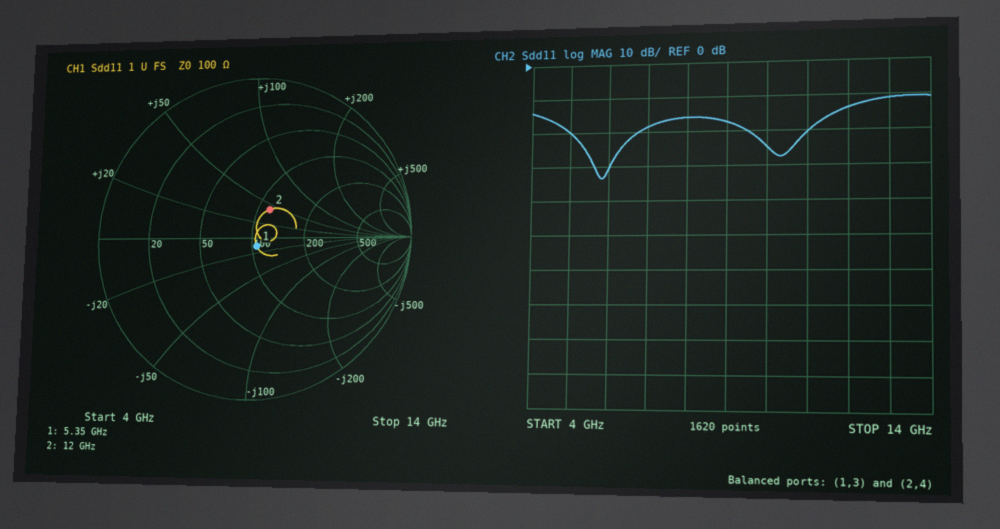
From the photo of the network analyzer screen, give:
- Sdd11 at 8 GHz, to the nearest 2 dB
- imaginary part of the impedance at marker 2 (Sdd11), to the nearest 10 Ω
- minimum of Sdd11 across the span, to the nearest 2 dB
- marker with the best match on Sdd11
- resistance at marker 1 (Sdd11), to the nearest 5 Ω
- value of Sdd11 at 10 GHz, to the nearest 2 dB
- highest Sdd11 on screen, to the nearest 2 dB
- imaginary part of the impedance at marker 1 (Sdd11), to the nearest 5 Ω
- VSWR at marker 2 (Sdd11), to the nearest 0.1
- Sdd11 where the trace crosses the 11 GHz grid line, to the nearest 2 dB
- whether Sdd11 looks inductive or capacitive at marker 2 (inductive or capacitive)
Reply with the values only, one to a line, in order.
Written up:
-16 dB
+40 Ω
-34 dB
marker 1
105 Ω
-24 dB
-10 dB
-10 Ω
1.5
-20 dB
inductive
